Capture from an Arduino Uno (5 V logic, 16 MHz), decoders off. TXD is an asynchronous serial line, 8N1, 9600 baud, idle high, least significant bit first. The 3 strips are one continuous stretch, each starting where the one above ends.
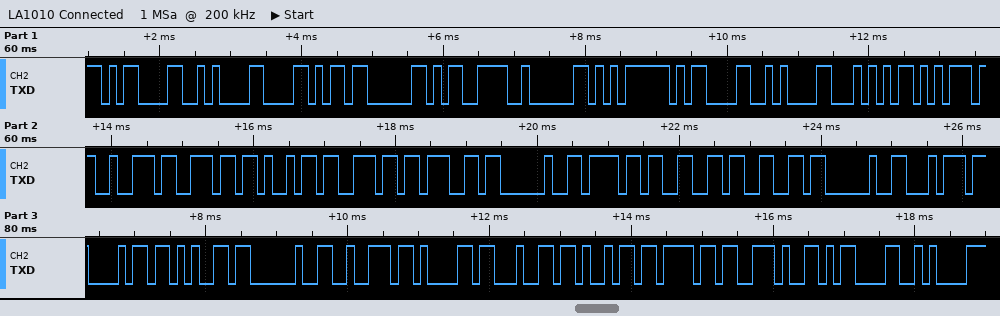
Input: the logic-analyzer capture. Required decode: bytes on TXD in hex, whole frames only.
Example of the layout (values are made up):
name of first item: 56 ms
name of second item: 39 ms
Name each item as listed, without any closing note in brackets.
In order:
bytes on TXD in hex, whole frames only: 0D 0A 58 03 CD 02 F5 0D 0A 54 75 72 6E 69 6E 67 20 6F 66 66 20 74 68 65 20 72 61 64 69 6F 2E 0D 0A
